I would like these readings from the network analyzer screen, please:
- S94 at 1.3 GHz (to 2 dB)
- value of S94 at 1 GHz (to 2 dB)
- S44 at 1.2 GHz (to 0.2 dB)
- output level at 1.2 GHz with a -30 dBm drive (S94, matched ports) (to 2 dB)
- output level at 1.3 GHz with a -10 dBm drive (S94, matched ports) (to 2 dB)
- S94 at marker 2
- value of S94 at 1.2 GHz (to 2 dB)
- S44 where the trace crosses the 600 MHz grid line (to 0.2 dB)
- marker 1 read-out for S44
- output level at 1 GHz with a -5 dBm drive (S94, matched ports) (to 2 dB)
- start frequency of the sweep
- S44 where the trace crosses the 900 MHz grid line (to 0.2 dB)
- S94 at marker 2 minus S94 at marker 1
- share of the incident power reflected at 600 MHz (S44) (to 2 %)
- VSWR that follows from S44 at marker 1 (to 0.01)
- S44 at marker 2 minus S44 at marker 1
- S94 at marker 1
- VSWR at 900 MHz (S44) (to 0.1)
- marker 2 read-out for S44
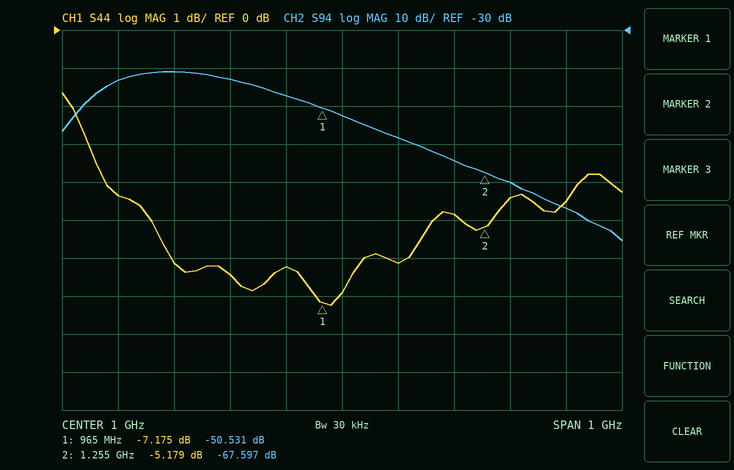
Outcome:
-70 dB
-52 dB
-4.8 dB
-94 dBm
-80 dBm
-67.597 dB
-64 dB
-4.4 dB
-7.175 dB
-58 dBm
500 MHz
-6.2 dB
-17.066 dB
36 %
2.56
1.996 dB
-50.531 dB
2.9
-5.179 dB
